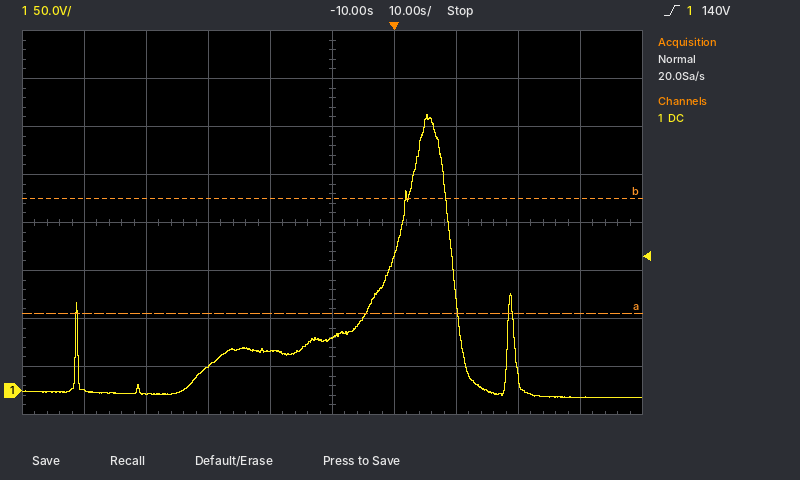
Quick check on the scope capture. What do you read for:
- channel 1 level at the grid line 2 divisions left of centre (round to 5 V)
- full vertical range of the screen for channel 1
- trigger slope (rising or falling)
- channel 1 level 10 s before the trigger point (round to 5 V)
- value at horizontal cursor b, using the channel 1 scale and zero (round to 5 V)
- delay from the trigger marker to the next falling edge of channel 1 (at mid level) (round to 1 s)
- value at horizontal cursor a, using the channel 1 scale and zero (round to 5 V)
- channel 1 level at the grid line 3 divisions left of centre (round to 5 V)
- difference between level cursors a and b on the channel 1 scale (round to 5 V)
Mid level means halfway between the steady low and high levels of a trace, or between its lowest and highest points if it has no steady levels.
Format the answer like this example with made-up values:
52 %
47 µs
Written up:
25 V
400 V
rising
55 V
200 V
9 s
80 V
-5 V
120 V
